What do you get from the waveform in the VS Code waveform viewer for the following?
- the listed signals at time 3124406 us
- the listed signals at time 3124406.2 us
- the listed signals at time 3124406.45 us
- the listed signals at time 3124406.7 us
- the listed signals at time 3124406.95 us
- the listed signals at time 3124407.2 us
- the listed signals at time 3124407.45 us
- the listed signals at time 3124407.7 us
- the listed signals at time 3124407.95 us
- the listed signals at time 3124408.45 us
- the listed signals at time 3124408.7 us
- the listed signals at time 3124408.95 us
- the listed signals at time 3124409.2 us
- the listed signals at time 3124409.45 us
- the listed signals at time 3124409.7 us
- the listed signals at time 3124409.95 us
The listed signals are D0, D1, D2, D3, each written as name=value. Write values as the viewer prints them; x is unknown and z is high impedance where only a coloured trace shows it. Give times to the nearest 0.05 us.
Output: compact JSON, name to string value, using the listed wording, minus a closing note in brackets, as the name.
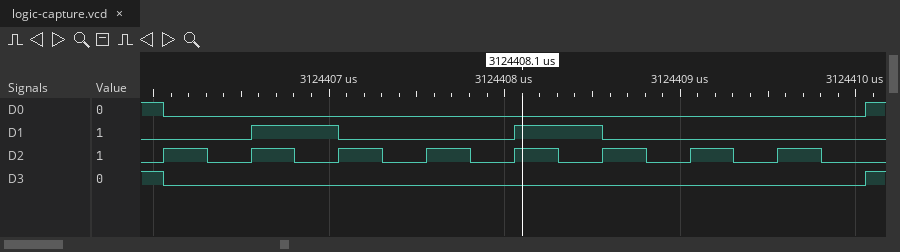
{"the listed signals at time 3124406 us": "D0=1, D1=0, D2=0, D3=1", "the listed signals at time 3124406.2 us": "D0=0, D1=0, D2=1, D3=0", "the listed signals at time 3124406.45 us": "D0=0, D1=0, D2=0, D3=0", "the listed signals at time 3124406.7 us": "D0=0, D1=1, D2=1, D3=0", "the listed signals at time 3124406.95 us": "D0=0, D1=1, D2=0, D3=0", "the listed signals at time 3124407.2 us": "D0=0, D1=0, D2=1, D3=0", "the listed signals at time 3124407.45 us": "D0=0, D1=0, D2=0, D3=0", "the listed signals at time 3124407.7 us": "D0=0, D1=0, D2=1, D3=0", "the listed signals at time 3124407.95 us": "D0=0, D1=0, D2=0, D3=0", "the listed signals at time 3124408.45 us": "D0=0, D1=1, D2=0, D3=0", "the listed signals at time 3124408.7 us": "D0=0, D1=0, D2=1, D3=0", "the listed signals at time 3124408.95 us": "D0=0, D1=0, D2=0, D3=0", "the listed signals at time 3124409.2 us": "D0=0, D1=0, D2=1, D3=0", "the listed signals at time 3124409.45 us": "D0=0, D1=0, D2=0, D3=0", "the listed signals at time 3124409.7 us": "D0=0, D1=0, D2=1, D3=0", "the listed signals at time 3124409.95 us": "D0=0, D1=0, D2=0, D3=0"}
